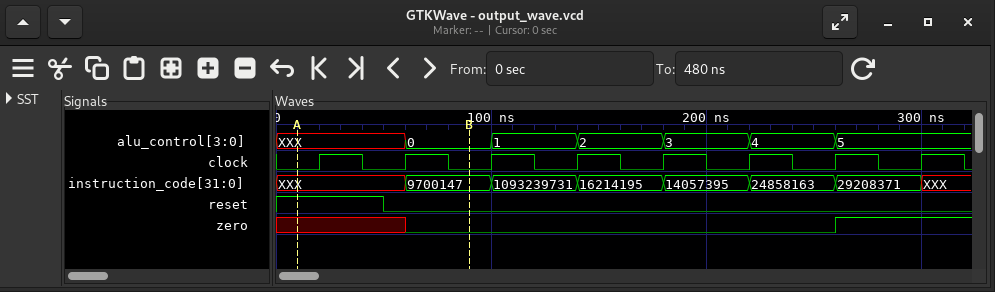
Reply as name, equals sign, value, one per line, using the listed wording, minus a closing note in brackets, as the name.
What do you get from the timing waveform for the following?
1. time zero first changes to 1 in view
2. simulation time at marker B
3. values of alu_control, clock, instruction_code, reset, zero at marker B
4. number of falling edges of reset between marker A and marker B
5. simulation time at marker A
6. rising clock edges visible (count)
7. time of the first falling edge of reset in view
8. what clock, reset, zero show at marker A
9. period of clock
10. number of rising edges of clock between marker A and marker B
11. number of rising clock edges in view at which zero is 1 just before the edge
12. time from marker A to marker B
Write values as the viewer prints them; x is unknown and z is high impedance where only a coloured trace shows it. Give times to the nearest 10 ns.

time zero first changes to 1 in view = 260 ns
simulation time at marker B = 90 ns
values of alu_control, clock, instruction_code, reset, zero at marker B = alu_control=0, clock=0, instruction_code=9700147, reset=0, zero=0
number of falling edges of reset between marker A and marker B = 1
simulation time at marker A = 10 ns
rising clock edges visible = 8
time of the first falling edge of reset in view = 50 ns
what clock, reset, zero show at marker A = clock=0, reset=1, zero=x
period of clock = 40 ns
number of rising edges of clock between marker A and marker B = 2
number of rising clock edges in view at which zero is 1 just before the edge = 1
time from marker A to marker B = 80 ns
